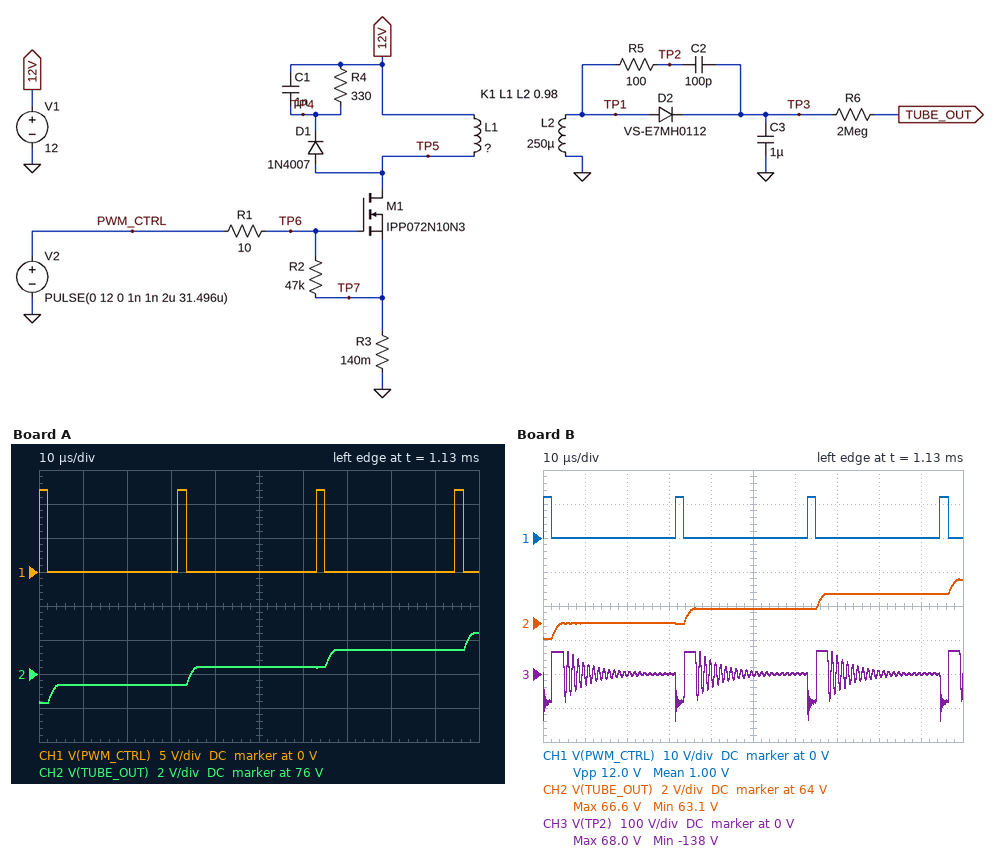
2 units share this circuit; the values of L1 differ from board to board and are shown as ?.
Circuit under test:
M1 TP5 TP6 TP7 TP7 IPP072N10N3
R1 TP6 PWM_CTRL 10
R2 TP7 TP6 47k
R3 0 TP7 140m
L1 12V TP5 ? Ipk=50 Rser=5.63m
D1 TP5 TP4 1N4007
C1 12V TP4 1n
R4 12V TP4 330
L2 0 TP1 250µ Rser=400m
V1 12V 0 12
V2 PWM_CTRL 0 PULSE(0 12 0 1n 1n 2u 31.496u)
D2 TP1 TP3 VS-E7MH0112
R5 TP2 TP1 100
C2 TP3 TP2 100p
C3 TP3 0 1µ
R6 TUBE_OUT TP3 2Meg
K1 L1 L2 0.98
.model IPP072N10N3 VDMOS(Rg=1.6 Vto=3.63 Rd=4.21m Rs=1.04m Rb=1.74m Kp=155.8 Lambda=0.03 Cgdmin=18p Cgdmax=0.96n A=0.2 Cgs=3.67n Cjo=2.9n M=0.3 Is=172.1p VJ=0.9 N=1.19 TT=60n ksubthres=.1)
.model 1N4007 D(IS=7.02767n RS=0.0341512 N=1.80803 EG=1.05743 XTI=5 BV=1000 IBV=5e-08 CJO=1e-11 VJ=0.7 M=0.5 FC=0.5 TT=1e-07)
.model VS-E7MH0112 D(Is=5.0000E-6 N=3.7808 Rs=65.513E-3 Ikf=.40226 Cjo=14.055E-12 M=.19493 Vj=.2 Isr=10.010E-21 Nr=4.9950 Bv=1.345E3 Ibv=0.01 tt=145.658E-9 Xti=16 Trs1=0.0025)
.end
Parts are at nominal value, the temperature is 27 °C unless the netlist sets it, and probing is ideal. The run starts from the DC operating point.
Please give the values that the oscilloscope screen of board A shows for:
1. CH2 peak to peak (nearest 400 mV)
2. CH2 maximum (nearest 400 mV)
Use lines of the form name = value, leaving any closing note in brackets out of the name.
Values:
CH2 peak to peak = 4.0 V
CH2 maximum = 78.4 V
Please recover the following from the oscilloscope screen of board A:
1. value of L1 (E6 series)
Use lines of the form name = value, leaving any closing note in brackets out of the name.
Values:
value of L1 = 3.3 µH
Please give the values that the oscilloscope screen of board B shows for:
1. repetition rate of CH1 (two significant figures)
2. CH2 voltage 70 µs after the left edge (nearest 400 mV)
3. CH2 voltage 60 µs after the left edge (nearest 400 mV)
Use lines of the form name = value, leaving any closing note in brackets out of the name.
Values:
repetition rate of CH1 = 32 kHz
CH2 voltage 70 µs after the left edge = 65.6 V
CH2 voltage 60 µs after the left edge = 64.8 V
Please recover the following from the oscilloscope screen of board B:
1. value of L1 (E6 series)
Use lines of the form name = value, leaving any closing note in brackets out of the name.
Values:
value of L1 = 4.7 µH
